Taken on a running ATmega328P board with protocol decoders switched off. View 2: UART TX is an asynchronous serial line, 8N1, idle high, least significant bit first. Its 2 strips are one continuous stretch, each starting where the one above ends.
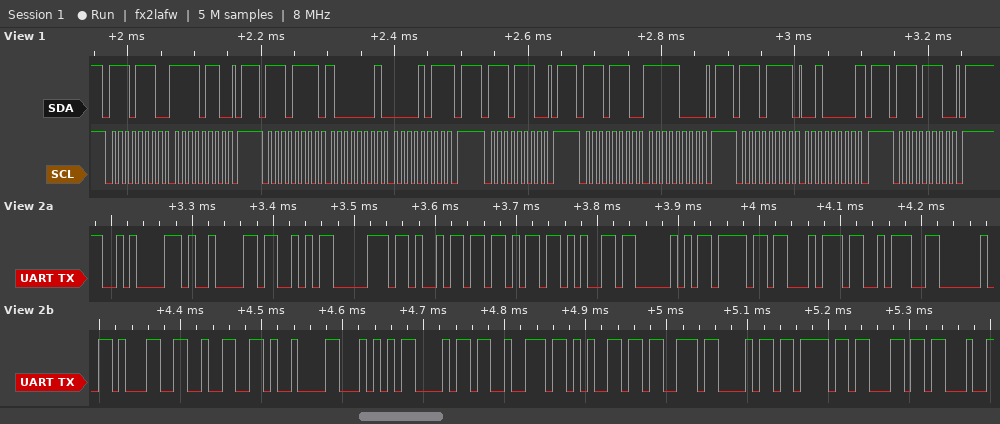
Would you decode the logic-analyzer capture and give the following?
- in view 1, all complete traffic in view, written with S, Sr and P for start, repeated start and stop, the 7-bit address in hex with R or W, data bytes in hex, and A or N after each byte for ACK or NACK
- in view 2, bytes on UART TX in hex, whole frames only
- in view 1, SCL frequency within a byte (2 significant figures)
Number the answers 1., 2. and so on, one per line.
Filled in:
1. S 77W A F6 A P S 77R A 81 A 0B N P S 77W A P S 77W A F8 A P S 77R A 20 N P S 77W A P
2. 0A 09 53 70 69 6B 65 50 6F 74 3A 20 31 32 09 54 68 72 65 73 68 6F 6C
3. 100 kHz
